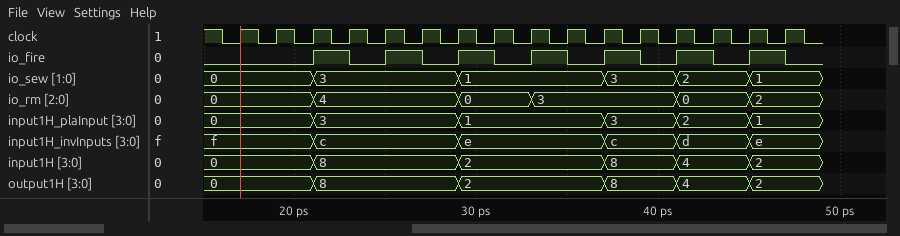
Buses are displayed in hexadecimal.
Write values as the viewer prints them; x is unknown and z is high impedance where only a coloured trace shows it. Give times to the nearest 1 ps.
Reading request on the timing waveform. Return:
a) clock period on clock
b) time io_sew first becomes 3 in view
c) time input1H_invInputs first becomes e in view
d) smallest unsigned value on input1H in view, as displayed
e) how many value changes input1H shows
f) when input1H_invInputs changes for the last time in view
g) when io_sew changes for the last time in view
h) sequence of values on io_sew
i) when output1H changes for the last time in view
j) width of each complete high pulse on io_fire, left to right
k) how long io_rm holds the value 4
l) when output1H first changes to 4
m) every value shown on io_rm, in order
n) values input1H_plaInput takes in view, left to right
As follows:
2 ps
21 ps
29 ps
0
5
45 ps
45 ps
0, 3, 1, 3, 2, 1
45 ps
2 ps, 2 ps, 2 ps, 2 ps, 2 ps, 2 ps, 2 ps
8 ps
41 ps
0, 4, 0, 3, 0, 2
0, 3, 1, 3, 2, 1
